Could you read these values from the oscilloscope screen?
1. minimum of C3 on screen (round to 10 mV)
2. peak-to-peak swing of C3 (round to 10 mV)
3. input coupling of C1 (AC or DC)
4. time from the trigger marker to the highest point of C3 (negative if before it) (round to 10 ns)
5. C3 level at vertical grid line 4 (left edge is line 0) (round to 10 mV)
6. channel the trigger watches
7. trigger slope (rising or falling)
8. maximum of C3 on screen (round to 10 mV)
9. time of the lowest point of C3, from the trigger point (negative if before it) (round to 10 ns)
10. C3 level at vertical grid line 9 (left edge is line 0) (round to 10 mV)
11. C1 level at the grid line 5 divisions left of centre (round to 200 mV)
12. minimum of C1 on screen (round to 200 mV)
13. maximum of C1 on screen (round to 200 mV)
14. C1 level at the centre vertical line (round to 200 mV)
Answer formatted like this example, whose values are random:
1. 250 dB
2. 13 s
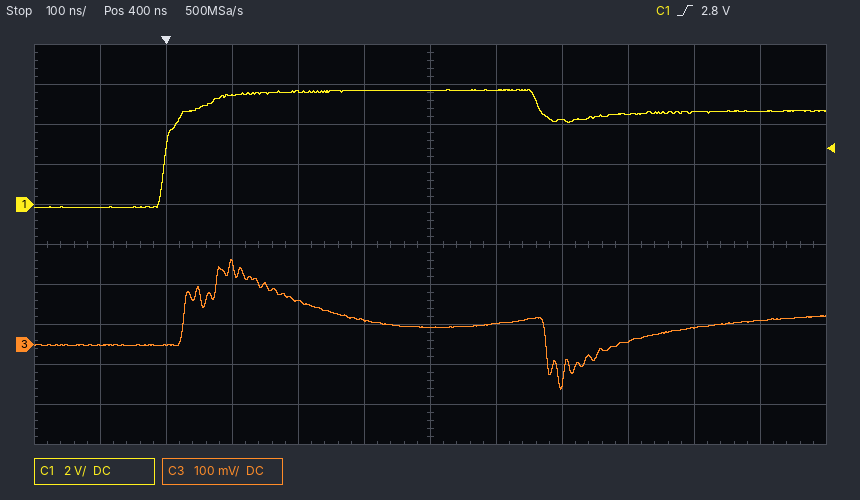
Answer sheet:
1. -110 mV
2. 320 mV
3. DC
4. +100 ns
5. 110 mV
6. C1
7. rising
8. 210 mV
9. +600 ns
10. 10 mV
11. -200 mV
12. -200 mV
13. 5.8 V
14. 5.6 V
